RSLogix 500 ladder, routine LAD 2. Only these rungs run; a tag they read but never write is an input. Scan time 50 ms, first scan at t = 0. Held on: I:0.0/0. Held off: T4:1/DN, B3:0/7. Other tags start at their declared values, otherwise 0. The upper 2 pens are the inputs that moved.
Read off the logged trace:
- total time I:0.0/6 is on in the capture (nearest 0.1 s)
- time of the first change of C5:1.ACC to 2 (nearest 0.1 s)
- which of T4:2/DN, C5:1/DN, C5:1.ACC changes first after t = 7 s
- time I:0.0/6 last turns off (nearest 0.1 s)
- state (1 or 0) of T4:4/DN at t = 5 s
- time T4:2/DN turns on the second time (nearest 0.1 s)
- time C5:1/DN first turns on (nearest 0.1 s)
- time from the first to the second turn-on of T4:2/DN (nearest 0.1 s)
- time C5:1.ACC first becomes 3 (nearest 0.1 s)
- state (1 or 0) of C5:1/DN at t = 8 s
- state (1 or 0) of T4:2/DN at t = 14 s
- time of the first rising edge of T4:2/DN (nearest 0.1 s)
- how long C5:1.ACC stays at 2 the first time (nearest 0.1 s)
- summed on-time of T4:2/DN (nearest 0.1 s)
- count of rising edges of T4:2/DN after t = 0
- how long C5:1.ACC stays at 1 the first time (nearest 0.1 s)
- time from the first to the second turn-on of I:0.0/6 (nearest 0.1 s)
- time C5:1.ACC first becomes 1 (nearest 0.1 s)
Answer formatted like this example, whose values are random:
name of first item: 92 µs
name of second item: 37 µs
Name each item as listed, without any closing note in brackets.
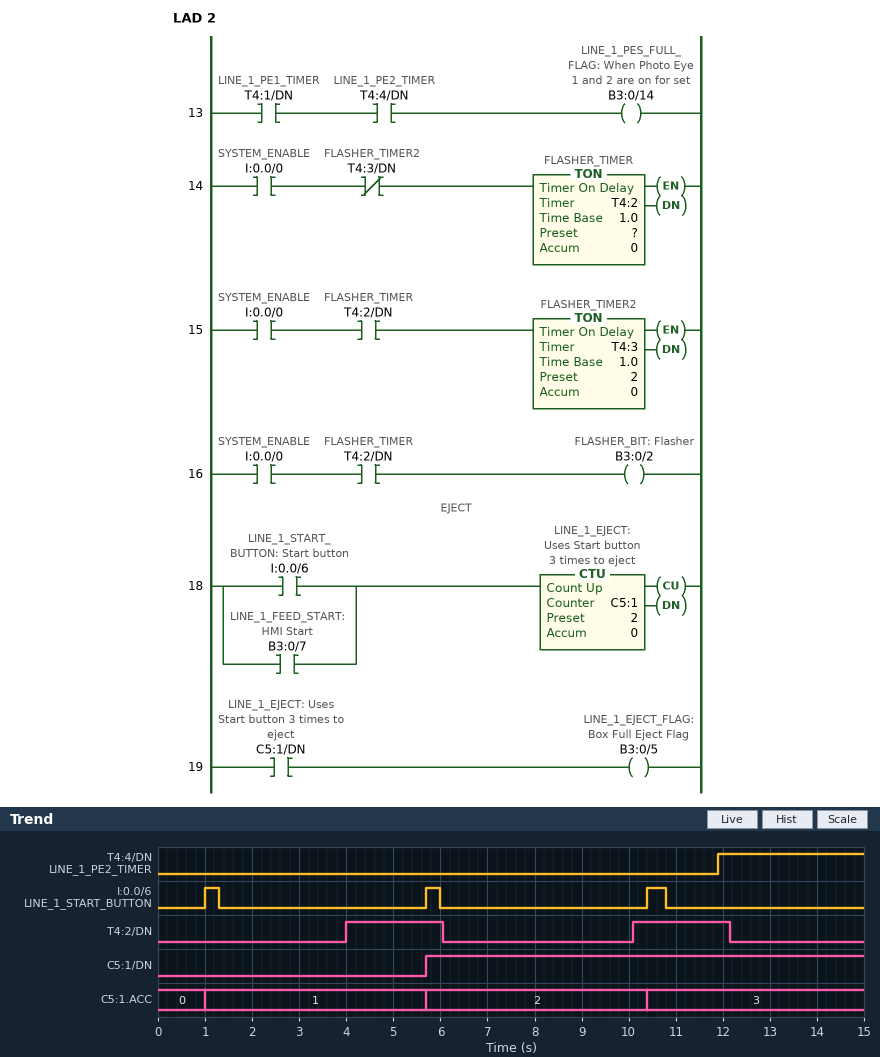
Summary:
total time I:0.0/6 is on in the capture: 1.0 s
time of the first change of C5:1.ACC to 2: 5.7 s
which of T4:2/DN, C5:1/DN, C5:1.ACC changes first after t = 7 s: T4:2/DN
time I:0.0/6 last turns off: 10.8 s
state (1 or 0) of T4:4/DN at t = 5 s: 0
time T4:2/DN turns on the second time: 10.1 s
time C5:1/DN first turns on: 5.7 s
time from the first to the second turn-on of T4:2/DN: 6.1 s
time C5:1.ACC first becomes 3: 10.4 s
state (1 or 0) of C5:1/DN at t = 8 s: 1
state (1 or 0) of T4:2/DN at t = 14 s: 0
time of the first rising edge of T4:2/DN: 4.0 s
how long C5:1.ACC stays at 2 the first time: 4.7 s
summed on-time of T4:2/DN: 4.1 s
count of rising edges of T4:2/DN after t = 0: 2
how long C5:1.ACC stays at 1 the first time: 4.7 s
time from the first to the second turn-on of I:0.0/6: 4.7 s
time C5:1.ACC first becomes 1: 1.0 s
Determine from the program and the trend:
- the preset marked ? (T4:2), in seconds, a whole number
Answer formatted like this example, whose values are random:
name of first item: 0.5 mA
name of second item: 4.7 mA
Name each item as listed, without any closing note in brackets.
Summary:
the preset marked ? (T4:2), in seconds, a whole number: 4 s
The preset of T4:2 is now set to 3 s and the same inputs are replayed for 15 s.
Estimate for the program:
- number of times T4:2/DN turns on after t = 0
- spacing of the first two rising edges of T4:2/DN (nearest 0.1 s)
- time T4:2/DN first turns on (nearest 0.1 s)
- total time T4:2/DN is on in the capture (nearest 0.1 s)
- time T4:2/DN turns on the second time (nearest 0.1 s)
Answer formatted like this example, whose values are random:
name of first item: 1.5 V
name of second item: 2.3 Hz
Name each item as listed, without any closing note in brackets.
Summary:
number of times T4:2/DN turns on after t = 0: 3
spacing of the first two rising edges of T4:2/DN: 5.1 s
time T4:2/DN first turns on: 3.0 s
total time T4:2/DN is on in the capture: 5.9 s
time T4:2/DN turns on the second time: 8.1 s
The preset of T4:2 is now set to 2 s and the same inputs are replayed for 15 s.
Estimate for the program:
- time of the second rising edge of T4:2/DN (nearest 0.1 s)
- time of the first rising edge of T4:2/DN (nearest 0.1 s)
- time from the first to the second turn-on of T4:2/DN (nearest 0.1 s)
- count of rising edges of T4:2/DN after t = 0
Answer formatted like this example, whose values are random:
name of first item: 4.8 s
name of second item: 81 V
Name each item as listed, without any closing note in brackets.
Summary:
time of the second rising edge of T4:2/DN: 6.1 s
time of the first rising edge of T4:2/DN: 2.0 s
time from the first to the second turn-on of T4:2/DN: 4.1 s
count of rising edges of T4:2/DN after t = 0: 4
